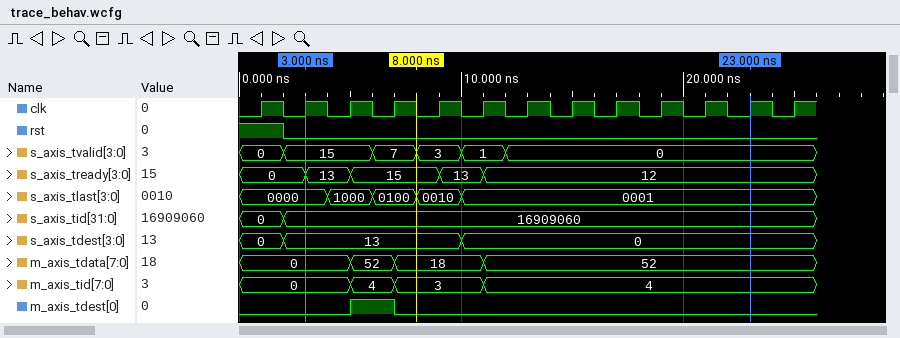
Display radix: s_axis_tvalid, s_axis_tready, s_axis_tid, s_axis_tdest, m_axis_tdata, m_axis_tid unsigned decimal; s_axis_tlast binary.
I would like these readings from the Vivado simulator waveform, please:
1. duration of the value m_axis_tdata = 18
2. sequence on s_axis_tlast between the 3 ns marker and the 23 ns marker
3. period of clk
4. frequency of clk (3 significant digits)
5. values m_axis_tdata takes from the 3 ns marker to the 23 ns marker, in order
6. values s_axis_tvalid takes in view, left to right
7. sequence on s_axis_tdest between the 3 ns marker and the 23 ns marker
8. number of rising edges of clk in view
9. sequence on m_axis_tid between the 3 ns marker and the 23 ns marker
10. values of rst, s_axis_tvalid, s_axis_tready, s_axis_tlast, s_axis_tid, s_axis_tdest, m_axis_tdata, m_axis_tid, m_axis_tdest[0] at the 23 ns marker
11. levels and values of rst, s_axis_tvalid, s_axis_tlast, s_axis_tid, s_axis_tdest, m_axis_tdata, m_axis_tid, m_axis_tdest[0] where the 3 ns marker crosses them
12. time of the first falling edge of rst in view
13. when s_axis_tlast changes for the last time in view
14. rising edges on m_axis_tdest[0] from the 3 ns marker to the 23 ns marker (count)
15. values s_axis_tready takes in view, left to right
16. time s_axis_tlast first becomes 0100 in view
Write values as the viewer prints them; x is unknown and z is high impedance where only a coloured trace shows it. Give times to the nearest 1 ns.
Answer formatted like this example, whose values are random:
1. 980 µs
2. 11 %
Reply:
1. 4 ns
2. 0000, 1000, 0100, 0010, 0001
3. 2 ns
4. 500 MHz
5. 0, 52, 18, 52
6. 0, 15, 7, 3, 1, 0
7. 13, 0
8. 13
9. 0, 4, 3, 4
10. rst=0, s_axis_tvalid=0, s_axis_tready=12, s_axis_tlast=0001, s_axis_tid=16909060, s_axis_tdest=0, m_axis_tdata=52, m_axis_tid=4, m_axis_tdest[0]=0
11. rst=0, s_axis_tvalid=15, s_axis_tlast=0000, s_axis_tid=16909060, s_axis_tdest=13, m_axis_tdata=0, m_axis_tid=0, m_axis_tdest[0]=0
12. 2 ns
13. 10 ns
14. 1
15. 0, 13, 15, 13, 12
16. 6 ns
